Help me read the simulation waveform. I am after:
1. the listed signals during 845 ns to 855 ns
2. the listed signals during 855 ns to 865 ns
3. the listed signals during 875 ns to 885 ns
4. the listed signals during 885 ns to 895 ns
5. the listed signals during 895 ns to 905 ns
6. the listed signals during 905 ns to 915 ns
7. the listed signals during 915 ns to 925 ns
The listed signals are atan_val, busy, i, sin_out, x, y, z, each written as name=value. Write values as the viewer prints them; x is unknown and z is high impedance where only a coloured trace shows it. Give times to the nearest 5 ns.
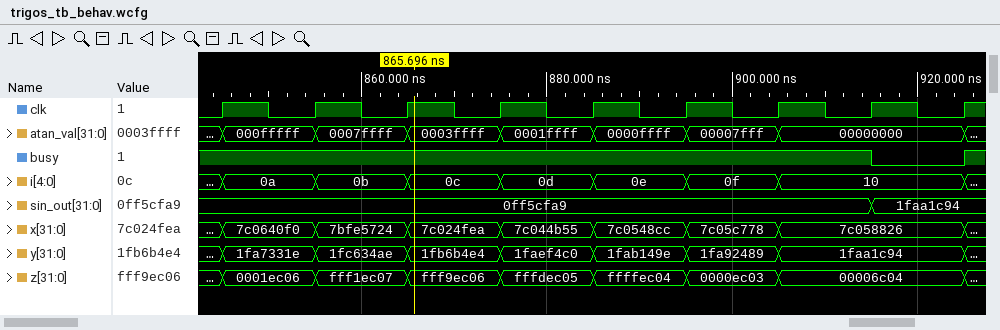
atan_val=000fffff, busy=1, i=0a, sin_out=0ff5cfa9, x=7c0640f0, y=1fa7331e, z=0001ec06
atan_val=0007ffff, busy=1, i=0b, sin_out=0ff5cfa9, x=7bfe5724, y=1fc634ae, z=fff1ec07
atan_val=0001ffff, busy=1, i=0d, sin_out=0ff5cfa9, x=7c044b55, y=1faef4c0, z=fffdec05
atan_val=0000ffff, busy=1, i=0e, sin_out=0ff5cfa9, x=7c0548cc, y=1fab149e, z=ffffec04
atan_val=00007fff, busy=1, i=0f, sin_out=0ff5cfa9, x=7c05c778, y=1fa92489, z=0000ec03
atan_val=00000000, busy=1, i=10, sin_out=0ff5cfa9, x=7c058826, y=1faa1c94, z=00006c04
atan_val=00000000, busy=0, i=10, sin_out=1faa1c94, x=7c058826, y=1faa1c94, z=00006c04
